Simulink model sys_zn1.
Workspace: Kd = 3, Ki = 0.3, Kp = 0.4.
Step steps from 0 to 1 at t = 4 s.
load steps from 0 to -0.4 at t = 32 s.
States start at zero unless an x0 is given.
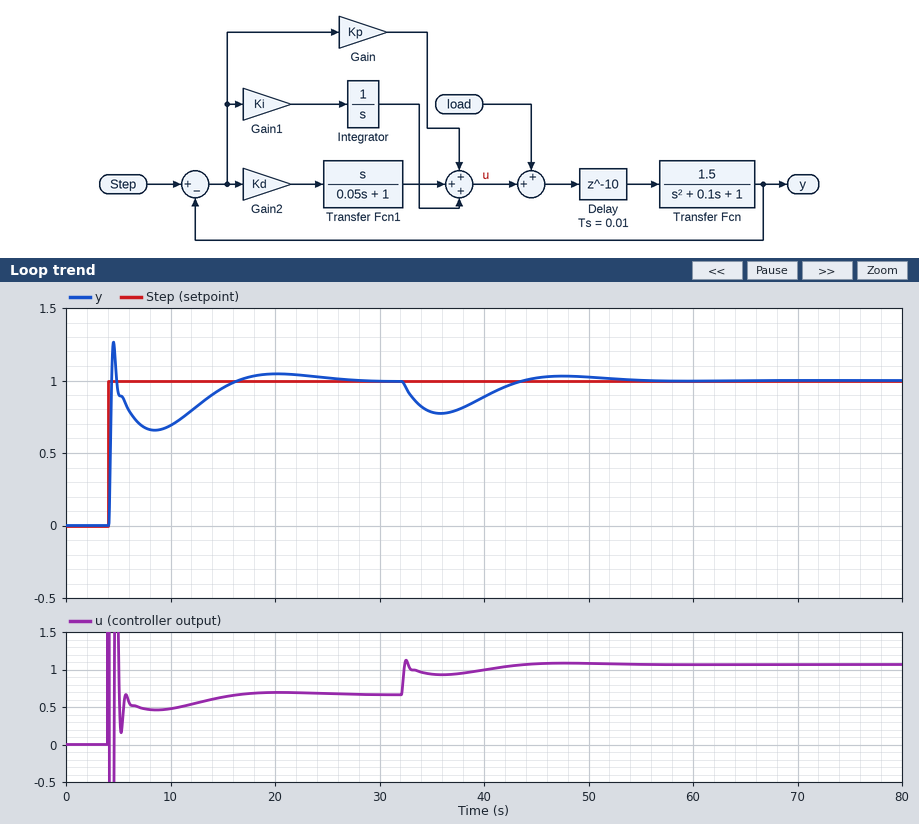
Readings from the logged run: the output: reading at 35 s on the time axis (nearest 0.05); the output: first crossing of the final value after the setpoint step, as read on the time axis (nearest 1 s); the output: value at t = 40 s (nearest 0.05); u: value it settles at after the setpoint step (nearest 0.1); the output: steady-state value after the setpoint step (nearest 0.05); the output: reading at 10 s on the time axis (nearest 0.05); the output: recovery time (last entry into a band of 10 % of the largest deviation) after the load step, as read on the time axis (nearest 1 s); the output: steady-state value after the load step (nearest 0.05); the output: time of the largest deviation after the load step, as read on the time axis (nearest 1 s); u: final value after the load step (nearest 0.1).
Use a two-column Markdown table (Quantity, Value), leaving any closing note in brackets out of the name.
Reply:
| Quantity | Value |
|---|---|
| the output: reading at 35 s on the time axis | 0.80 |
| the output: first crossing of the final value after the setpoint step, as read on the time axis | 4 s |
| the output: value at t = 40 s | 0.90 |
| u: value it settles at after the setpoint step | 0.7 |
| the output: steady-state value after the setpoint step | 1.00 |
| the output: reading at 10 s on the time axis | 0.70 |
| the output: recovery time (last entry into a band of 10 % of the largest deviation) after the load step, as read on the time axis | 50 s |
| the output: steady-state value after the load step | 1.00 |
| the output: time of the largest deviation after the load step, as read on the time axis | 36 s |
| u: final value after the load step | 1.1 |
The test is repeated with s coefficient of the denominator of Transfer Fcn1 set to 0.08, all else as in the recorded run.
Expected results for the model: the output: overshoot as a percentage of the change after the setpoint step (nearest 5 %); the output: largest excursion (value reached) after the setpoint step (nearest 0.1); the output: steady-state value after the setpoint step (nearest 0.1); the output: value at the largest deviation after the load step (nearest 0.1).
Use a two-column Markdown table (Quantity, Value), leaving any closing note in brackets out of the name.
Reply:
| Quantity | Value |
|---|---|
| the output: overshoot as a percentage of the change after the setpoint step | 30 % |
| the output: largest excursion (value reached) after the setpoint step | 1.3 |
| the output: steady-state value after the setpoint step | 1.0 |
| the output: value at the largest deviation after the load step | 0.8 |
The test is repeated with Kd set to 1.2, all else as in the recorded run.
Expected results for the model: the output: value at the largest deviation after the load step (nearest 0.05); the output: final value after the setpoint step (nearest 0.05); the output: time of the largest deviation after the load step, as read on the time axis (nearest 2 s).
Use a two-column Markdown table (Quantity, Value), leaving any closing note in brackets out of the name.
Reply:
| Quantity | Value |
|---|---|
| the output: value at the largest deviation after the load step | 0.70 |
| the output: final value after the setpoint step | 1.00 |
| the output: time of the largest deviation after the load step, as read on the time axis | 34 s |
